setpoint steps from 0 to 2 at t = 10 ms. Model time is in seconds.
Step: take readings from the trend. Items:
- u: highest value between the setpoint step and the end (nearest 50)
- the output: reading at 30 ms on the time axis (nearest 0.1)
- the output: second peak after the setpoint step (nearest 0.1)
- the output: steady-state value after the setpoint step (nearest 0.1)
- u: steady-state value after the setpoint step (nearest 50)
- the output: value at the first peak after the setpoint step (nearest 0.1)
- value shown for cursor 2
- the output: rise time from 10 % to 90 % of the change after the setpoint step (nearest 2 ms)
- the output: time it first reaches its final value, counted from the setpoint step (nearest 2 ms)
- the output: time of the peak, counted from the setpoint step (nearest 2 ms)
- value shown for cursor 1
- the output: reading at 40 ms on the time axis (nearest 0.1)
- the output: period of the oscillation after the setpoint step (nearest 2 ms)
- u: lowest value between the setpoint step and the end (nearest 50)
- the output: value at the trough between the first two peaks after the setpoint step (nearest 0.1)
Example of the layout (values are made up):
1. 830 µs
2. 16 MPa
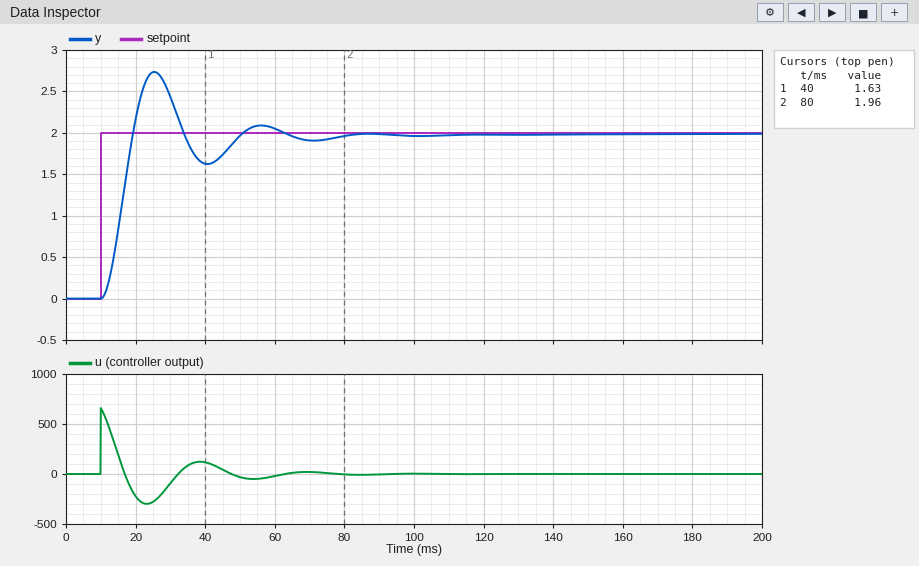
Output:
1. 650
2. 2.4
3. 2.1
4. 2.0
5. 0
6. 2.7
7. 1.96
8. 6 ms
9. 10 ms
10. 16 ms
11. 1.63
12. 1.6
13. 30 ms
14. -300
15. 1.6
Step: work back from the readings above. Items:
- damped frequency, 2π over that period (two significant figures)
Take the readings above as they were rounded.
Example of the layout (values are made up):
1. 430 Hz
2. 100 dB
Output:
1. 0.21 rad/ms
